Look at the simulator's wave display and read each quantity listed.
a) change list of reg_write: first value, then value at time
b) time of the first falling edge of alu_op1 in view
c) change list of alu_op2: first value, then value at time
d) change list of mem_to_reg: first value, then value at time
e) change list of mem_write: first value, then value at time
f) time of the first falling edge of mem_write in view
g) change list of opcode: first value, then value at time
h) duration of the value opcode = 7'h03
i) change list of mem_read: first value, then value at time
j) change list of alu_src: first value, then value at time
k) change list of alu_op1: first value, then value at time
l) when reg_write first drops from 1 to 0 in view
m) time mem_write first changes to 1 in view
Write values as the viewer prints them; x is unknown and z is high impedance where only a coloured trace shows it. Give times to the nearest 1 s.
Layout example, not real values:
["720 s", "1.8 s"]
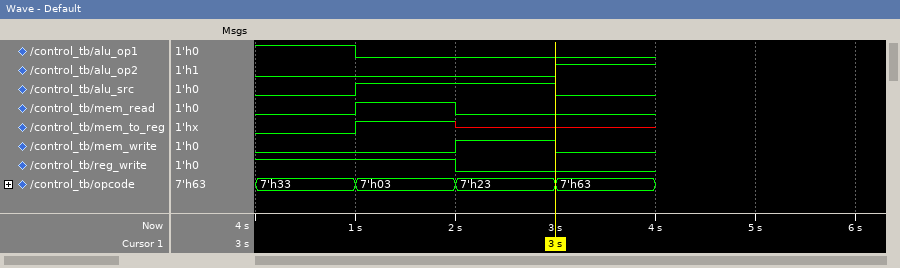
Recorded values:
["1, 0 at 2 s", "1 s", "0, 1 at 3 s", "0, 1 at 1 s, x at 2 s", "0, 1 at 2 s, 0 at 3 s", "3 s", "7'h33, 7'h03 at 1 s, 7'h23 at 2 s, 7'h63 at 3 s", "1 s", "0, 1 at 1 s, 0 at 2 s", "0, 1 at 1 s, 0 at 3 s", "1, 0 at 1 s", "2 s", "2 s"]
